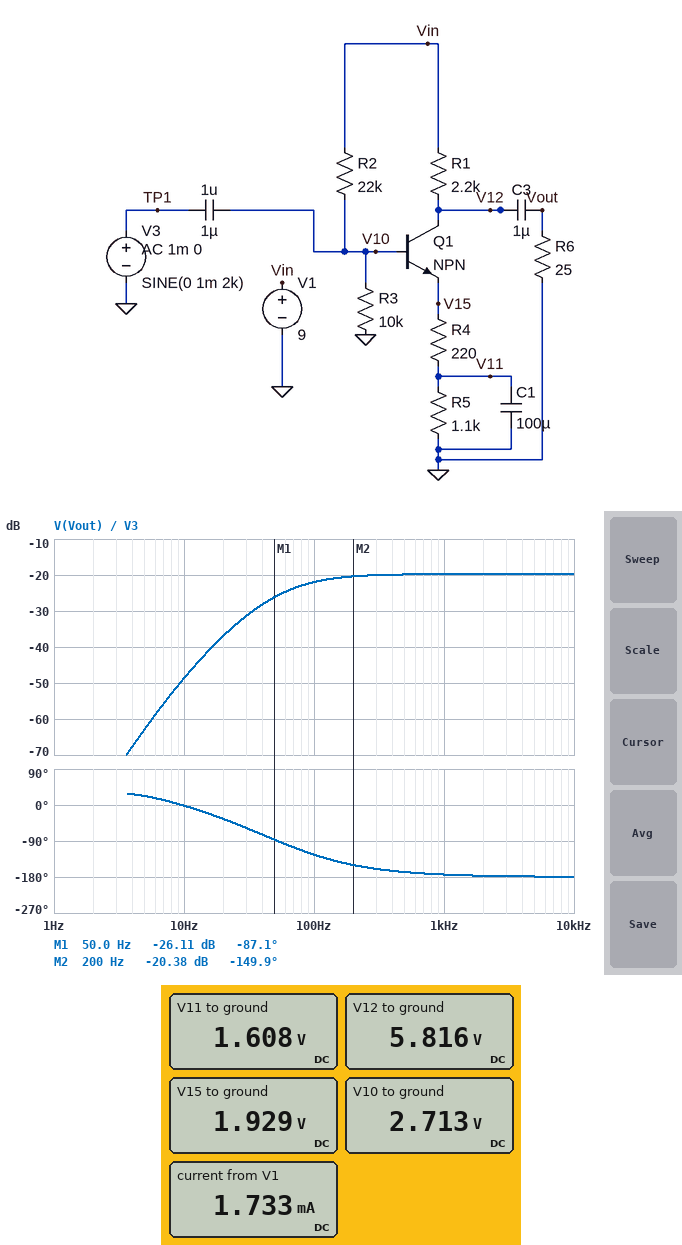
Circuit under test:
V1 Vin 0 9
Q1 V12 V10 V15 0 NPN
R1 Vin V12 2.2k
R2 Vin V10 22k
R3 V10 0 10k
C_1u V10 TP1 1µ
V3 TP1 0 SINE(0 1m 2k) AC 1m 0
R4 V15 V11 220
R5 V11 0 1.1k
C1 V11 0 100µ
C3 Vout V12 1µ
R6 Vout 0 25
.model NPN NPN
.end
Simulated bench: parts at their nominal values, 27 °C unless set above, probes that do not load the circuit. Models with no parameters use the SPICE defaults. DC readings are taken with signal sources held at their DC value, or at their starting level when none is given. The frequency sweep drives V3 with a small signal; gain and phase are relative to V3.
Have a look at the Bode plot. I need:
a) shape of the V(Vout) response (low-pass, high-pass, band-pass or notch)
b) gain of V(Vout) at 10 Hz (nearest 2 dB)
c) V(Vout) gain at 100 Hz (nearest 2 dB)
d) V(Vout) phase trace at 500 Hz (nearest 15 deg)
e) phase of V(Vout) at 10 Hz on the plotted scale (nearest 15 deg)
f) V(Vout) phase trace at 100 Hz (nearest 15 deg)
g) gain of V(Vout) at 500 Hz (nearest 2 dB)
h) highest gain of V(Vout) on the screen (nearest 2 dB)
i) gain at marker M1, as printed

high-pass
-48 dB
-22 dB
-165 deg
0 deg
-120 deg
-20 dB
-20 dB
-26.11 dB
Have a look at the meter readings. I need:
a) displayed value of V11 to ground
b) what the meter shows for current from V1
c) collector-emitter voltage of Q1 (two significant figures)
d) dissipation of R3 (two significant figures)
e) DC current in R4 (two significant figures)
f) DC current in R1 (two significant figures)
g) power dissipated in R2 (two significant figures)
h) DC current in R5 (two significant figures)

1.608 V
1.733 mA
3.9 V
740 µW
1.5 mA
1.4 mA
1.8 mW
1.5 mA
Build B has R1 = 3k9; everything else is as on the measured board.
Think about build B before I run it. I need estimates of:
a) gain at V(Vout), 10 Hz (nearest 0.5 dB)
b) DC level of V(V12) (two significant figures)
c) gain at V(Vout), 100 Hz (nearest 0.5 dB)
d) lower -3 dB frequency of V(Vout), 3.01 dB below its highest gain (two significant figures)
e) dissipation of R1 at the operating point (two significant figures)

-44.0 dB
3.4 V
-21.0 dB
57 Hz
8.2 mW
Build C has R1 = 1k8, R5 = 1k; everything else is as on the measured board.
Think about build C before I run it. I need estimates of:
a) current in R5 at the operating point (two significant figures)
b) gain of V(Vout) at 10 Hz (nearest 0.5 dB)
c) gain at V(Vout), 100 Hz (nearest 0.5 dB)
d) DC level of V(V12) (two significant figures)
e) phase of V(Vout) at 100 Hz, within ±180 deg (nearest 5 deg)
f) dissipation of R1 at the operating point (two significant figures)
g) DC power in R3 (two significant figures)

1.6 mA
-50.5 dB
-22.5 dB
6.2 V
-120 deg
4.4 mW
730 µW
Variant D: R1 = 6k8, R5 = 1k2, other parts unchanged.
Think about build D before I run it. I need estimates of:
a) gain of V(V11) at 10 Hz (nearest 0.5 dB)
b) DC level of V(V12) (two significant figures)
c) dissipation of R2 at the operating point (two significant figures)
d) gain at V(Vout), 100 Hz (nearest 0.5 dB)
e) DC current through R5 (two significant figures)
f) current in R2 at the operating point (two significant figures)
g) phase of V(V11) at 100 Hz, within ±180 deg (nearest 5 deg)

-40.5 dB
1.7 V
2.0 mW
-53.0 dB
1.1 mA
300 µA
0 deg
